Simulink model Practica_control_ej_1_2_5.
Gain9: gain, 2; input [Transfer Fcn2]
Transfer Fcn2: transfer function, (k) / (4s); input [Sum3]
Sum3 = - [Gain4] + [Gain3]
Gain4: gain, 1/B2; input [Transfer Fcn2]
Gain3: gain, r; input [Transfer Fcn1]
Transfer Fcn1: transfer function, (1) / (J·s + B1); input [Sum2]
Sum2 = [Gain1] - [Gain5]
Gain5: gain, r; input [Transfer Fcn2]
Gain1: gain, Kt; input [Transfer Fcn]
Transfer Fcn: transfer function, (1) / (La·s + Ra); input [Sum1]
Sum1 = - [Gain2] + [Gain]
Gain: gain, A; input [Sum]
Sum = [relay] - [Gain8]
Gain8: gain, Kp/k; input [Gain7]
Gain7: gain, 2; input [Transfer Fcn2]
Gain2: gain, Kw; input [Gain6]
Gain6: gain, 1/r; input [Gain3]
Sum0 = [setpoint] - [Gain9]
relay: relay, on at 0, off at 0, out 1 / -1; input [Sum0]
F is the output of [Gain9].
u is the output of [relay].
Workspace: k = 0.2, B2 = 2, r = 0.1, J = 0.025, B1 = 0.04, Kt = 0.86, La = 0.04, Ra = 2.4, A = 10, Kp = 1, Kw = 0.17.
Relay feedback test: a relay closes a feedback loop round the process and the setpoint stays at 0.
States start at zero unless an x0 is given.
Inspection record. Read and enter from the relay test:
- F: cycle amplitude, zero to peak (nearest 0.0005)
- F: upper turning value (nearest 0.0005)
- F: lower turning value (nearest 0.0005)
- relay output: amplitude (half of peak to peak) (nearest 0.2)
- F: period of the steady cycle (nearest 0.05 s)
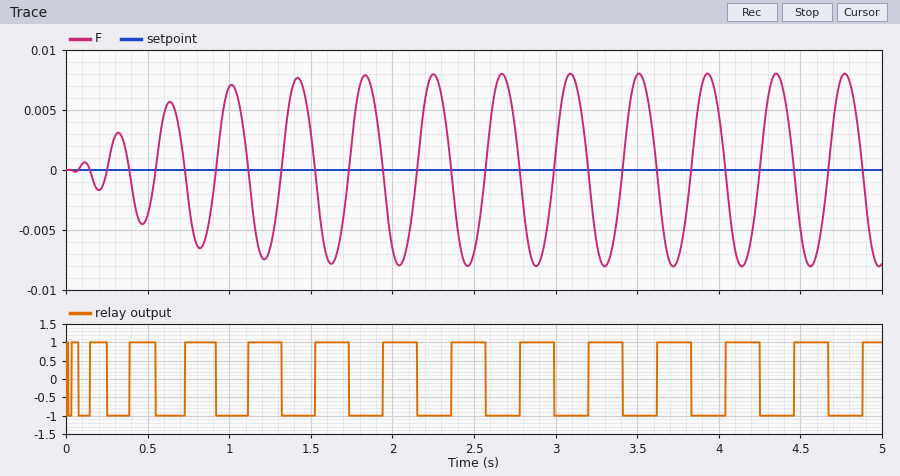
0.0080
0.0080
-0.0080
1.0
0.40 s
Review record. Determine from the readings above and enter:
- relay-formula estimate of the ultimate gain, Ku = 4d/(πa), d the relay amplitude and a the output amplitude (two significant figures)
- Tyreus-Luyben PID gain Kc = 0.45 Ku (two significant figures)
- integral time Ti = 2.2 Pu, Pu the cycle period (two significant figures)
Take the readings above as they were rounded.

160
72
0.88 s
